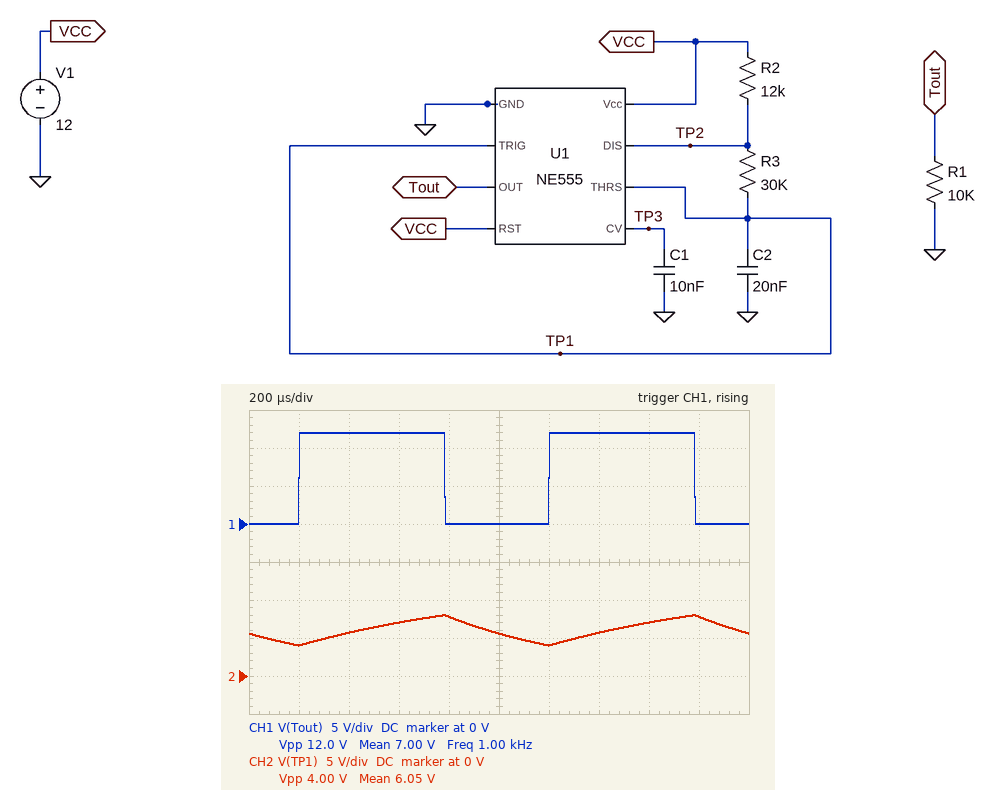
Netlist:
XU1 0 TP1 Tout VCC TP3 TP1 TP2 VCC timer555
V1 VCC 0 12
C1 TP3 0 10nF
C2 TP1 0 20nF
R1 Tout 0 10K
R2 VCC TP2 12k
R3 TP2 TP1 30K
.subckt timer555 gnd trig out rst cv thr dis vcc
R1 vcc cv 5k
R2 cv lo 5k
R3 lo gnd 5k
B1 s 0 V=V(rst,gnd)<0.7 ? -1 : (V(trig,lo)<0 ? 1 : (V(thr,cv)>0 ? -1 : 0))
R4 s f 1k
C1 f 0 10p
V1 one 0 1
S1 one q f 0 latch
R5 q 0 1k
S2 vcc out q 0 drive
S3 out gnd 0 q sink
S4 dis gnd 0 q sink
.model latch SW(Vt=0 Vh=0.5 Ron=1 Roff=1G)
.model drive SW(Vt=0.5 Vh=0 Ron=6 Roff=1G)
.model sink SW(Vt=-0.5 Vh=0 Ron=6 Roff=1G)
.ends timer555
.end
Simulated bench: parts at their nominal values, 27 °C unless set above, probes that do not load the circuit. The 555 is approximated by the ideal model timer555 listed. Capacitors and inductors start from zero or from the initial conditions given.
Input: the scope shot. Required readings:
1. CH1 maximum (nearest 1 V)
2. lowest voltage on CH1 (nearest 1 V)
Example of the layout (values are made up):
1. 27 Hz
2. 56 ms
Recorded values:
1. 12 V
2. 0 V
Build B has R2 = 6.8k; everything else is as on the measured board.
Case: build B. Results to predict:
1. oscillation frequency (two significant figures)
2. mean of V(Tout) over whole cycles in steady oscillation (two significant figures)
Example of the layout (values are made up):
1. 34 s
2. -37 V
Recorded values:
1. 1.1 kHz
2. 6.6 V
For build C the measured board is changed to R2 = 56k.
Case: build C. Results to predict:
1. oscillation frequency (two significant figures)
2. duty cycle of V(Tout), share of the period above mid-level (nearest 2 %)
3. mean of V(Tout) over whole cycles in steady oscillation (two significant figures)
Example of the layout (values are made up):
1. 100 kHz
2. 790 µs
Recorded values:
1. 620 Hz
2. 74 %
3. 8.9 V
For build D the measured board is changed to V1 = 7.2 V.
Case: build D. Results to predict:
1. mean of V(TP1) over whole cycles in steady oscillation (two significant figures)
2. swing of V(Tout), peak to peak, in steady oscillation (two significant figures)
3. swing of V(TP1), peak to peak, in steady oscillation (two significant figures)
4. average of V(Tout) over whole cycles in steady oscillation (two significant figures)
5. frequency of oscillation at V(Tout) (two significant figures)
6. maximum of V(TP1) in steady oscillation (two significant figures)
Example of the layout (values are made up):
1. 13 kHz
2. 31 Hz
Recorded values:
1. 3.6 V
2. 7.2 V
3. 2.4 V
4. 4.2 V
5. 1.0 kHz
6. 4.8 V
